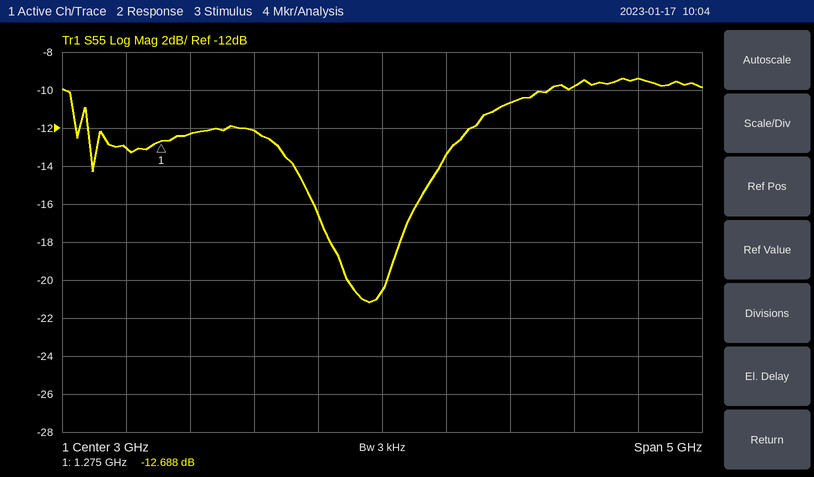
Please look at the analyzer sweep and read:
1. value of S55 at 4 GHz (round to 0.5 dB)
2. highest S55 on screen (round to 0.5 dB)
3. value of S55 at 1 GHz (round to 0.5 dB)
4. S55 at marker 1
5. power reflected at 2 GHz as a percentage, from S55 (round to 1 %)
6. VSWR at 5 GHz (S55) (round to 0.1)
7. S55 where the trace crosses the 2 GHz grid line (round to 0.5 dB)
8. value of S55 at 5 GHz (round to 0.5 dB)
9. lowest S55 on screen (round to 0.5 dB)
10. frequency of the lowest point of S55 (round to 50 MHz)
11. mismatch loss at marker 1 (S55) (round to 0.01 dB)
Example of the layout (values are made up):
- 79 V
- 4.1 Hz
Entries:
- -10.5 dB
- -9.5 dB
- -13.0 dB
- -12.688 dB
- 6 %
- 2.0
- -12.0 dB
- -9.5 dB
- -21.0 dB
- 2.90 GHz
- 0.24 dB
